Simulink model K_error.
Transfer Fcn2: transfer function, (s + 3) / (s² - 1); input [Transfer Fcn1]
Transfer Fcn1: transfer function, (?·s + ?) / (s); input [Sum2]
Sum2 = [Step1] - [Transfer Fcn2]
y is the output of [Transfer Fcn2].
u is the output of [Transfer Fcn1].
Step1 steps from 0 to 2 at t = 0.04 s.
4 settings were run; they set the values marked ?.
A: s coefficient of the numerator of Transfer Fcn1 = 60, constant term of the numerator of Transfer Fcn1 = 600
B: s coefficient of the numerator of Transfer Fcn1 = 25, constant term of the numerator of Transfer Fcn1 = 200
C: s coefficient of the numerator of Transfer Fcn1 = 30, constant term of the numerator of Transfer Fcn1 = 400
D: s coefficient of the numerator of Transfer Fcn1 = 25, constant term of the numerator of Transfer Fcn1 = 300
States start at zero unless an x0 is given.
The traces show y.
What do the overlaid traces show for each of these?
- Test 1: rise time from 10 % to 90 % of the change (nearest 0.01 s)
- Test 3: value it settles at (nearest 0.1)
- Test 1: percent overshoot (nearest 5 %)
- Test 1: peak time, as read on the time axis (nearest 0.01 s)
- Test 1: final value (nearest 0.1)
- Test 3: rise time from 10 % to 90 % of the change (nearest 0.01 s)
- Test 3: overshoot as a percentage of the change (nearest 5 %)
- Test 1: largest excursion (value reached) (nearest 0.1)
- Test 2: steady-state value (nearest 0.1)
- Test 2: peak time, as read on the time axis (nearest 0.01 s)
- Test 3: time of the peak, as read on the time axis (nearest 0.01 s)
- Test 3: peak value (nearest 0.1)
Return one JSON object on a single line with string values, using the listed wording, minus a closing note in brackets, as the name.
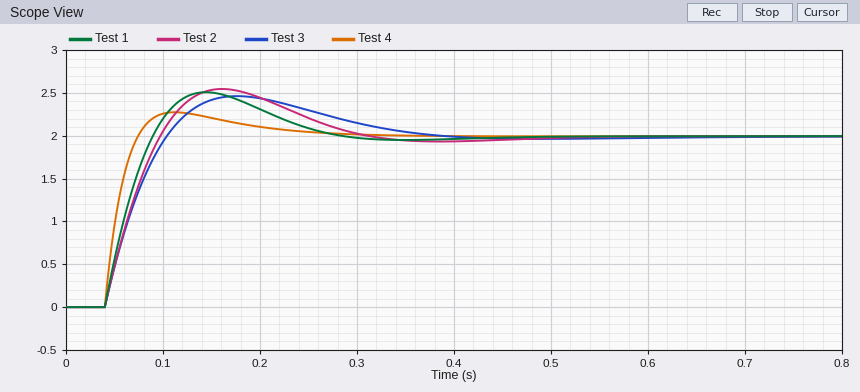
{"Test 1: rise time from 10 % to 90 % of the change": "0.04 s", "Test 3: value it settles at": "2.0", "Test 1: percent overshoot": "25 %", "Test 1: peak time, as read on the time axis": "0.14 s", "Test 1: final value": "2.0", "Test 3: rise time from 10 % to 90 % of the change": "0.05 s", "Test 3: overshoot as a percentage of the change": "25 %", "Test 1: largest excursion (value reached)": "2.5", "Test 2: steady-state value": "2.0", "Test 2: peak time, as read on the time axis": "0.16 s", "Test 3: time of the peak, as read on the time axis": "0.18 s", "Test 3: peak value": "2.5"}
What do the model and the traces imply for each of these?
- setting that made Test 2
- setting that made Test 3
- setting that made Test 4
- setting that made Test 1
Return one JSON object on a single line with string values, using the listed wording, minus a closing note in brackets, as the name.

{"setting that made Test 2": "D", "setting that made Test 3": "B", "setting that made Test 4": "A", "setting that made Test 1": "C"}
